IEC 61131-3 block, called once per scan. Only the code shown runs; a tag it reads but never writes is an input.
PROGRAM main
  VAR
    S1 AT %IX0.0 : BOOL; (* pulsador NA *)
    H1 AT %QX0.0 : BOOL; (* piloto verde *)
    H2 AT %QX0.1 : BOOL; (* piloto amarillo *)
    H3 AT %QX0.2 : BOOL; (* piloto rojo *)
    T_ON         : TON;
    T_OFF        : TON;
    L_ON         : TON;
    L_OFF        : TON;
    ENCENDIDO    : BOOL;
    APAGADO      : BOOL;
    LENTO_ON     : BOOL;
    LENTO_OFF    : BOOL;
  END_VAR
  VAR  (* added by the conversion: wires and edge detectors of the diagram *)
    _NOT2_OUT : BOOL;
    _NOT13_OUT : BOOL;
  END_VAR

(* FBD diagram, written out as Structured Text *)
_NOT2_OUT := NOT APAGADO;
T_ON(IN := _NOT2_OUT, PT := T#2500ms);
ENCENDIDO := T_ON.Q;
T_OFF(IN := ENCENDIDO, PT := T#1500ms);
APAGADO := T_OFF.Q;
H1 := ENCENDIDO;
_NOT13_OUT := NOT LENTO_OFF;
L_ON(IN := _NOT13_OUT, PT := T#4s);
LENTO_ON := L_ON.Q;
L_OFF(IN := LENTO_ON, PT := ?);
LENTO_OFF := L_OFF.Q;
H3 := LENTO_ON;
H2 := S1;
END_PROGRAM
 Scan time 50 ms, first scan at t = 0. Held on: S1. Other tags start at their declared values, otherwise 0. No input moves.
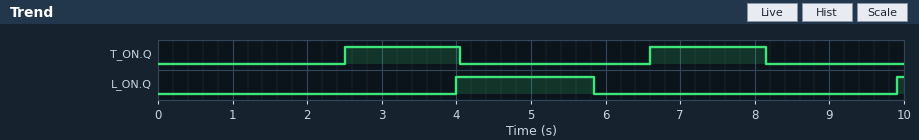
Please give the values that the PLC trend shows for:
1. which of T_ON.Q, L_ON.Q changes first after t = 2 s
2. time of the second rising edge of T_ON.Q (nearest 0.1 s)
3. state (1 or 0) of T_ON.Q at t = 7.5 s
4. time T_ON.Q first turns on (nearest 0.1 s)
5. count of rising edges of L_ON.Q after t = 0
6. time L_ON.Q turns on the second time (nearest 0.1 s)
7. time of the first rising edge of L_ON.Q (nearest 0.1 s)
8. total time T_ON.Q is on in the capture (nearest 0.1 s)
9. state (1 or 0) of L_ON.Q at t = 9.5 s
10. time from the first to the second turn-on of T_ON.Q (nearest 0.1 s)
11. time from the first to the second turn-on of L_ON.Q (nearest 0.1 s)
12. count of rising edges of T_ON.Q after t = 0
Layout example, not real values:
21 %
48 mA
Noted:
T_ON.Q
6.6 s
1
2.5 s
2
9.9 s
4.0 s
3.1 s
0
4.1 s
5.9 s
2
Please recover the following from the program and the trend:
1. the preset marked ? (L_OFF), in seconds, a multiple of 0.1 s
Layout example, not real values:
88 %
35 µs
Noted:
1.8 s
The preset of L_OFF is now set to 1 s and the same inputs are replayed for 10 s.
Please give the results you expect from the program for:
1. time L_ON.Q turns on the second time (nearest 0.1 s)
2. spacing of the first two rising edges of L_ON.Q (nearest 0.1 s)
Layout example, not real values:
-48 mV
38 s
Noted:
9.1 s
5.1 s
